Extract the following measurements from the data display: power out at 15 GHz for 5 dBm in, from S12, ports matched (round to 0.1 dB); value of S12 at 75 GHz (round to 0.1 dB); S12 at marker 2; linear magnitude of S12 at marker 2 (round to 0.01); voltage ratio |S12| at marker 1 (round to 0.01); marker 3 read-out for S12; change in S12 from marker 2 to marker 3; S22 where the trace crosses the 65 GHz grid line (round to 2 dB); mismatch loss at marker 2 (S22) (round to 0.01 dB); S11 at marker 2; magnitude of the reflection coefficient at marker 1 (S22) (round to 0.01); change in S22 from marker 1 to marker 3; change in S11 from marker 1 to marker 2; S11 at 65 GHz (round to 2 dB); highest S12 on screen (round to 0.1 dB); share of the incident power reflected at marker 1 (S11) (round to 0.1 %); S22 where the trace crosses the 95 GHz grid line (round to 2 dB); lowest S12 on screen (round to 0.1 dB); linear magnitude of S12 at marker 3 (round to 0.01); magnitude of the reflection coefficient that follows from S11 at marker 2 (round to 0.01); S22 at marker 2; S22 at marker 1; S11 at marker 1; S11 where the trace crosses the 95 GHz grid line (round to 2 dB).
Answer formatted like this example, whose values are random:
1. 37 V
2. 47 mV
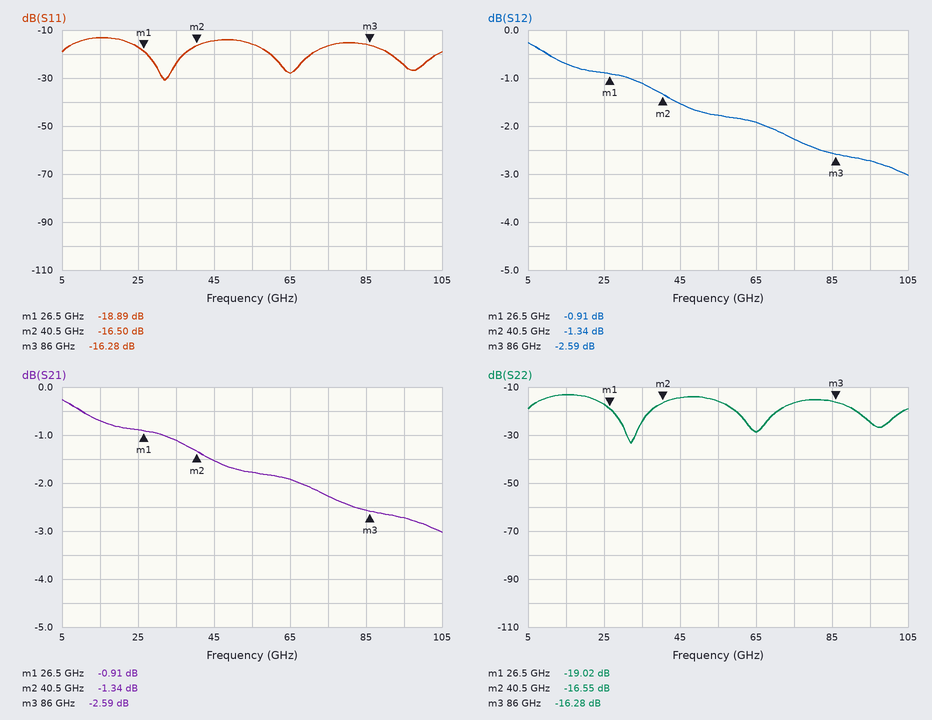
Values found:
1. 4.3 dBm
2. -2.3 dB
3. -1.34 dB
4. 0.86
5. 0.90
6. -2.59 dB
7. -1.25 dB
8. -28 dB
9. 0.10 dB
10. -16.50 dB
11. 0.11
12. 2.74 dB
13. 2.39 dB
14. -28 dB
15. -0.3 dB
16. 1.3 %
17. -24 dB
18. -3.0 dB
19. 0.74
20. 0.15
21. -16.55 dB
22. -19.02 dB
23. -18.89 dB
24. -24 dB
